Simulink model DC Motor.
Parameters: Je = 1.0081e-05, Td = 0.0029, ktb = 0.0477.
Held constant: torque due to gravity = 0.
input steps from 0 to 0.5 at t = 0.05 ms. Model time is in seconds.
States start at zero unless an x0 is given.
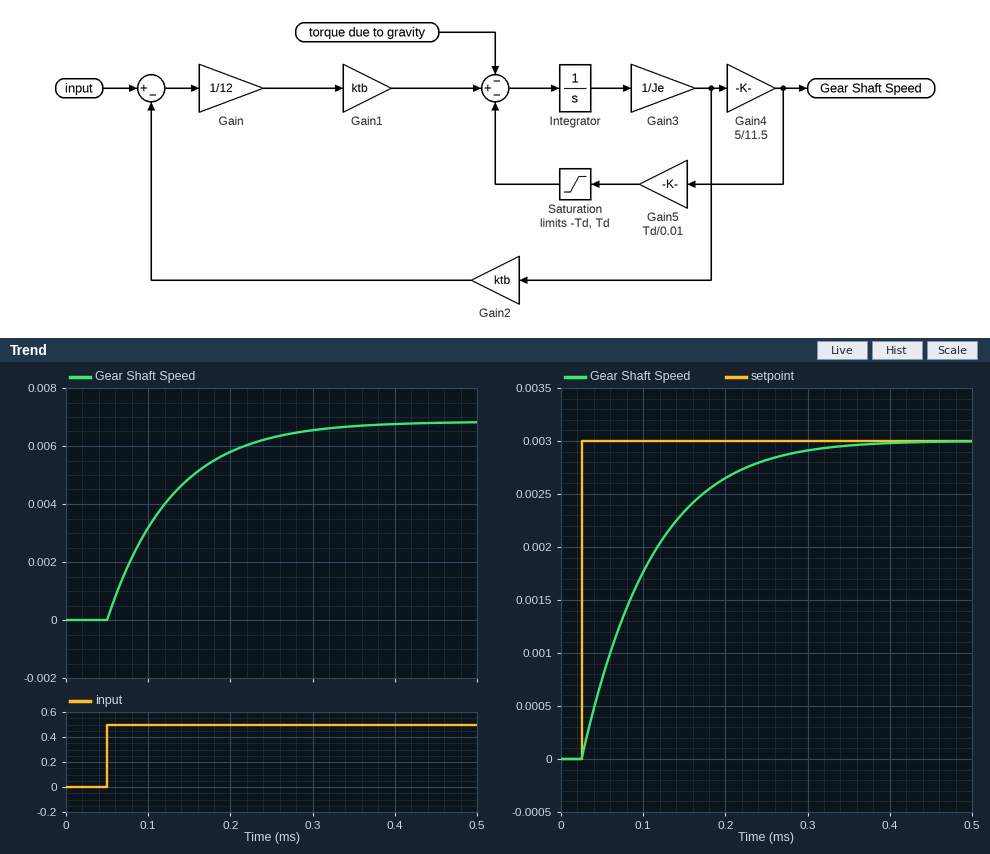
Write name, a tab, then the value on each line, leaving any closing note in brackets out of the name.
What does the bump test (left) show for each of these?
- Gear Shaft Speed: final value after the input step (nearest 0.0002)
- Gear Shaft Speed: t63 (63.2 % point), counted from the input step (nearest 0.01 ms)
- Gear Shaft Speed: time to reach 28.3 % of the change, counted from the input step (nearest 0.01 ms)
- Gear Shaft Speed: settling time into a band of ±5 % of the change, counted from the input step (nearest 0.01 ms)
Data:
Gear Shaft Speed: final value after the input step	0.0068
Gear Shaft Speed: t63 (63.2 % point), counted from the input step	0.08 ms
Gear Shaft Speed: time to reach 28.3 % of the change, counted from the input step	0.03 ms
Gear Shaft Speed: settling time into a band of ±5 % of the change, counted from the input step	0.24 ms
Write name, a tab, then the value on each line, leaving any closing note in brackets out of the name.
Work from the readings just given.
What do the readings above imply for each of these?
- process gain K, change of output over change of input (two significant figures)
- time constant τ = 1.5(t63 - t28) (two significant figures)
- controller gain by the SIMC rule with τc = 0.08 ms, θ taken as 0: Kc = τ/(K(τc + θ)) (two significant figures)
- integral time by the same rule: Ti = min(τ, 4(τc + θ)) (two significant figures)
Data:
process gain K, change of output over change of input	0.014
time constant τ = 1.5(t63 - t28)	0.075 ms
controller gain by the SIMC rule with τc = 0.08 ms, θ taken as 0: Kc = τ/(K(τc + θ))	67
integral time by the same rule: Ti = min(τ, 4(τc + θ))	0.075 ms
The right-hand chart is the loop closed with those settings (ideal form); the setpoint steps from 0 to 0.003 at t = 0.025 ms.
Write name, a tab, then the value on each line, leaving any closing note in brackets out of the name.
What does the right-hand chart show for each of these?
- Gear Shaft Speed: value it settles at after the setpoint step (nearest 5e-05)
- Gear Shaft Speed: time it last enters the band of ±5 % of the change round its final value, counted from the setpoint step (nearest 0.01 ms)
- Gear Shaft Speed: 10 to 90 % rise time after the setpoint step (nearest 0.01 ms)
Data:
Gear Shaft Speed: value it settles at after the setpoint step	0.00300
Gear Shaft Speed: time it last enters the band of ±5 % of the change round its final value, counted from the setpoint step	0.24 ms
Gear Shaft Speed: 10 to 90 % rise time after the setpoint step	0.18 ms
